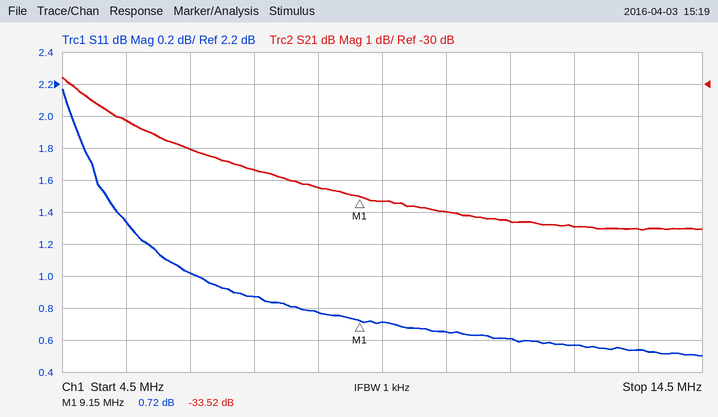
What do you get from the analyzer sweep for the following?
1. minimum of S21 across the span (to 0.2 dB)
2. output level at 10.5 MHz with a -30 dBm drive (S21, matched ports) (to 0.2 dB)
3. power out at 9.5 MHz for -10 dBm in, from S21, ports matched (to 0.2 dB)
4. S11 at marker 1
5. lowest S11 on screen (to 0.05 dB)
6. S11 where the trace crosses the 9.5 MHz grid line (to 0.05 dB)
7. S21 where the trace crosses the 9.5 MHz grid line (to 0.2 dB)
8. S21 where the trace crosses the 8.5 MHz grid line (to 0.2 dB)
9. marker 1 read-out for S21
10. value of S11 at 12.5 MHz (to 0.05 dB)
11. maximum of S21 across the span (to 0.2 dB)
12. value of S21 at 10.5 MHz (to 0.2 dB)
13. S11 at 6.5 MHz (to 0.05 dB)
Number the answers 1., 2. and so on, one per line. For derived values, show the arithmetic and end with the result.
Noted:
1. -34.6 dB
2. -30 dBm + (-34.0 dB) = -64.0 dBm
3. -10 dBm + (-33.6 dB) = -43.6 dBm
4. 0.72 dB
5. 0.50 dB
6. 0.70 dB
7. -33.6 dB
8. -33.2 dB
9. -33.52 dB
10. 0.55 dB
11. -29.8 dB
12. -34.0 dB
13. 1.00 dB
